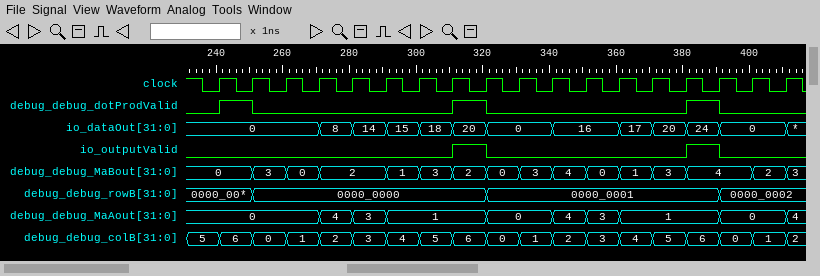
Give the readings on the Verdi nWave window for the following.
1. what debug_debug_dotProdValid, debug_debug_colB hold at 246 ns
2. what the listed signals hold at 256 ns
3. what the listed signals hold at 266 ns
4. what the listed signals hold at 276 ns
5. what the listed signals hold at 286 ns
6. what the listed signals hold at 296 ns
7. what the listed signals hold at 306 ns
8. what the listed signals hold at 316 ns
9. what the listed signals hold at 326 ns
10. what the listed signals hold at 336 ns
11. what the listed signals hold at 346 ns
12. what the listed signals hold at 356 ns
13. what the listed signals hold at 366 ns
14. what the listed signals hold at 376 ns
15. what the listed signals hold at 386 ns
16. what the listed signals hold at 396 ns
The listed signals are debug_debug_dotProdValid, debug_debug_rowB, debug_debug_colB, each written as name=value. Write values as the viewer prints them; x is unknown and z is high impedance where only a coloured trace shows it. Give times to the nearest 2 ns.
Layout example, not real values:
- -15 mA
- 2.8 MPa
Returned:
- debug_debug_dotProdValid=1, debug_debug_colB=6
- debug_debug_dotProdValid=0, debug_debug_rowB=0000_0000, debug_debug_colB=0
- debug_debug_dotProdValid=0, debug_debug_rowB=0000_0000, debug_debug_colB=1
- debug_debug_dotProdValid=0, debug_debug_rowB=0000_0000, debug_debug_colB=2
- debug_debug_dotProdValid=0, debug_debug_rowB=0000_0000, debug_debug_colB=3
- debug_debug_dotProdValid=0, debug_debug_rowB=0000_0000, debug_debug_colB=4
- debug_debug_dotProdValid=0, debug_debug_rowB=0000_0000, debug_debug_colB=5
- debug_debug_dotProdValid=1, debug_debug_rowB=0000_0000, debug_debug_colB=6
- debug_debug_dotProdValid=0, debug_debug_rowB=0000_0001, debug_debug_colB=0
- debug_debug_dotProdValid=0, debug_debug_rowB=0000_0001, debug_debug_colB=1
- debug_debug_dotProdValid=0, debug_debug_rowB=0000_0001, debug_debug_colB=2
- debug_debug_dotProdValid=0, debug_debug_rowB=0000_0001, debug_debug_colB=3
- debug_debug_dotProdValid=0, debug_debug_rowB=0000_0001, debug_debug_colB=4
- debug_debug_dotProdValid=0, debug_debug_rowB=0000_0001, debug_debug_colB=5
- debug_debug_dotProdValid=1, debug_debug_rowB=0000_0001, debug_debug_colB=6
- debug_debug_dotProdValid=0, debug_debug_rowB=0000_0002, debug_debug_colB=0
